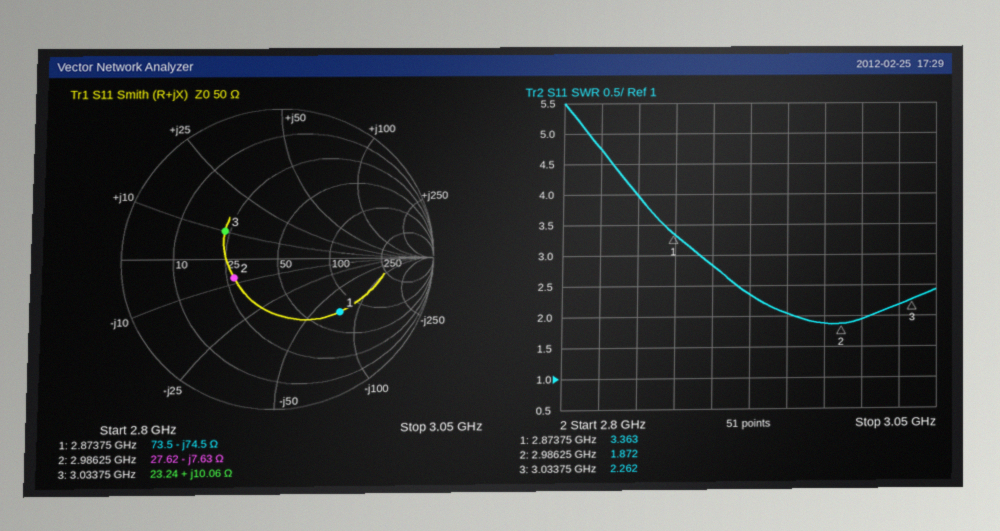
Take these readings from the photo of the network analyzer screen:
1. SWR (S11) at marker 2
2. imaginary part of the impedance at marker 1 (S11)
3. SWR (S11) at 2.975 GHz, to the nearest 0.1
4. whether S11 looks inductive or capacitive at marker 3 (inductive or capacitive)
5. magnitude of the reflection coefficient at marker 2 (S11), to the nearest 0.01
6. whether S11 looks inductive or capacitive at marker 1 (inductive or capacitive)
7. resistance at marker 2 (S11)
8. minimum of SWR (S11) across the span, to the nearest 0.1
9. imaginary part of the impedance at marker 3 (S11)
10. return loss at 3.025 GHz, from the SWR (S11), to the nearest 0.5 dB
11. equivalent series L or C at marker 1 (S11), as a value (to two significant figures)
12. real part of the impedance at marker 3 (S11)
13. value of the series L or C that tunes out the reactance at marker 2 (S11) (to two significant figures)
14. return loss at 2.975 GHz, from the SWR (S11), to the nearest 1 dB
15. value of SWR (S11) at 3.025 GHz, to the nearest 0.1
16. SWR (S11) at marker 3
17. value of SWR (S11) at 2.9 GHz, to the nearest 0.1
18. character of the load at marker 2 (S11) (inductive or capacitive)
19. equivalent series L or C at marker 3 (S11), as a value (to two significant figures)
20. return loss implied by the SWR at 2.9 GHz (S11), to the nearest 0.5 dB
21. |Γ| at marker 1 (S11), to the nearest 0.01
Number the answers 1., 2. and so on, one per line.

1. 1.872
2. -74.5 Ω
3. 1.9
4. inductive
5. 0.30
6. capacitive
7. 27.62 Ω
8. 1.9
9. +10.06 Ω
10. 8.5 dB
11. 740 fF
12. 23.24 Ω
13. 410 pH
14. 10 dB
15. 2.2
16. 2.262
17. 2.8
18. capacitive
19. 530 pH
20. 6.5 dB
21. 0.54
